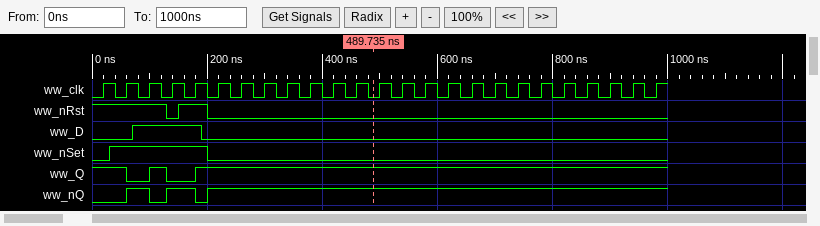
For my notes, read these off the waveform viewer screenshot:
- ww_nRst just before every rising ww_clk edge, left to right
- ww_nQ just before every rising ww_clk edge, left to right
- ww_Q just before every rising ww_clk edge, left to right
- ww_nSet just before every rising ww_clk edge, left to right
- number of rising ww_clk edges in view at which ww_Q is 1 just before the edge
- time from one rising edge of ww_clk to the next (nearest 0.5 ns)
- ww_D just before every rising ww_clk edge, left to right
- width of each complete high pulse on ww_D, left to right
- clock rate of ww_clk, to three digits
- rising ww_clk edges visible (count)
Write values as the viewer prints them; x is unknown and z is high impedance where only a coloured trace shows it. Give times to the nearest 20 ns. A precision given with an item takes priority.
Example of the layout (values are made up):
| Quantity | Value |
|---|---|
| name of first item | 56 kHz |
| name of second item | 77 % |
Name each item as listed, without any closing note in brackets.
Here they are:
| Quantity | Value |
|---|---|
| ww_nRst just before every rising ww_clk edge, left to right | 1 1 1 0 1 0 0 0 0 0 0 0 0 0 0 0 0 0 0 0 0 0 0 0 0 |
| ww_nQ just before every rising ww_clk edge, left to right | 0 0 1 1 1 1 1 1 1 1 1 1 1 1 1 1 1 1 1 1 1 1 1 1 1 |
| ww_Q just before every rising ww_clk edge, left to right | 1 1 0 0 0 1 1 1 1 1 1 1 1 1 1 1 1 1 1 1 1 1 1 1 1 |
| ww_nSet just before every rising ww_clk edge, left to right | 0 1 1 1 1 0 0 0 0 0 0 0 0 0 0 0 0 0 0 0 0 0 0 0 0 |
| number of rising ww_clk edges in view at which ww_Q is 1 just before the edge | 22 |
| time from one rising edge of ww_clk to the next | 40 ns |
| ww_D just before every rising ww_clk edge, left to right | 0 0 1 1 1 0 0 0 0 0 0 0 0 0 0 0 0 0 0 0 0 0 0 0 0 |
| width of each complete high pulse on ww_D, left to right | 120 ns |
| clock rate of ww_clk, to three digits | 25.0 MHz |
| rising ww_clk edges visible | 25 |
